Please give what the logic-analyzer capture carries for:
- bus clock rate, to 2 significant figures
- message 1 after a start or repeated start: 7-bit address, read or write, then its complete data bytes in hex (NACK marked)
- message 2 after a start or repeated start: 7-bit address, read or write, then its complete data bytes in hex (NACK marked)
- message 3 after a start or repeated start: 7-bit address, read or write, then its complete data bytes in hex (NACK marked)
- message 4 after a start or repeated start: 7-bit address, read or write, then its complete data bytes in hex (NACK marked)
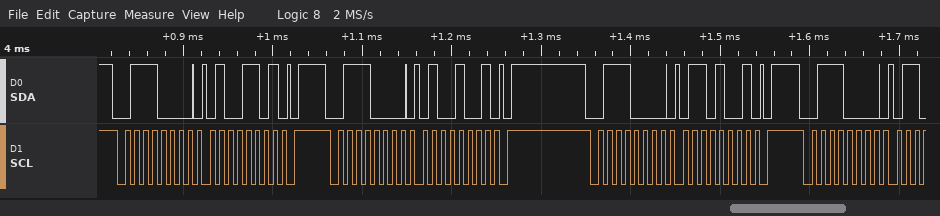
100 kHz
0x38 write: 4D
0x38 write: 49
0x38 write: 69
0x38 write
